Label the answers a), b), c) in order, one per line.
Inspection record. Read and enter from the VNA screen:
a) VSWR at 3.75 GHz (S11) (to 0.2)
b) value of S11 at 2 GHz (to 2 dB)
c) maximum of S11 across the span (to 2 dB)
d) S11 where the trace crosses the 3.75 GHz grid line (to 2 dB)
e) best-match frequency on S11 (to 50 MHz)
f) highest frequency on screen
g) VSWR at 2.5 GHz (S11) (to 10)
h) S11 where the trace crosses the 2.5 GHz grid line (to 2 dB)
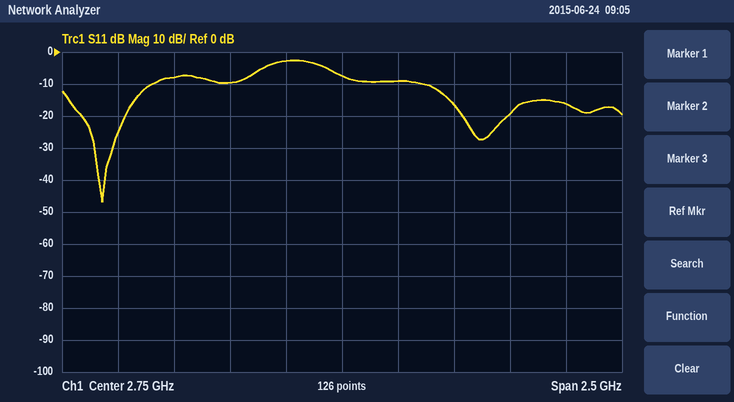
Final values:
a) 1.4
b) -8 dB
c) -2 dB
d) -16 dB
e) 1.70 GHz
f) 4 GHz
g) 10
h) -2 dB
